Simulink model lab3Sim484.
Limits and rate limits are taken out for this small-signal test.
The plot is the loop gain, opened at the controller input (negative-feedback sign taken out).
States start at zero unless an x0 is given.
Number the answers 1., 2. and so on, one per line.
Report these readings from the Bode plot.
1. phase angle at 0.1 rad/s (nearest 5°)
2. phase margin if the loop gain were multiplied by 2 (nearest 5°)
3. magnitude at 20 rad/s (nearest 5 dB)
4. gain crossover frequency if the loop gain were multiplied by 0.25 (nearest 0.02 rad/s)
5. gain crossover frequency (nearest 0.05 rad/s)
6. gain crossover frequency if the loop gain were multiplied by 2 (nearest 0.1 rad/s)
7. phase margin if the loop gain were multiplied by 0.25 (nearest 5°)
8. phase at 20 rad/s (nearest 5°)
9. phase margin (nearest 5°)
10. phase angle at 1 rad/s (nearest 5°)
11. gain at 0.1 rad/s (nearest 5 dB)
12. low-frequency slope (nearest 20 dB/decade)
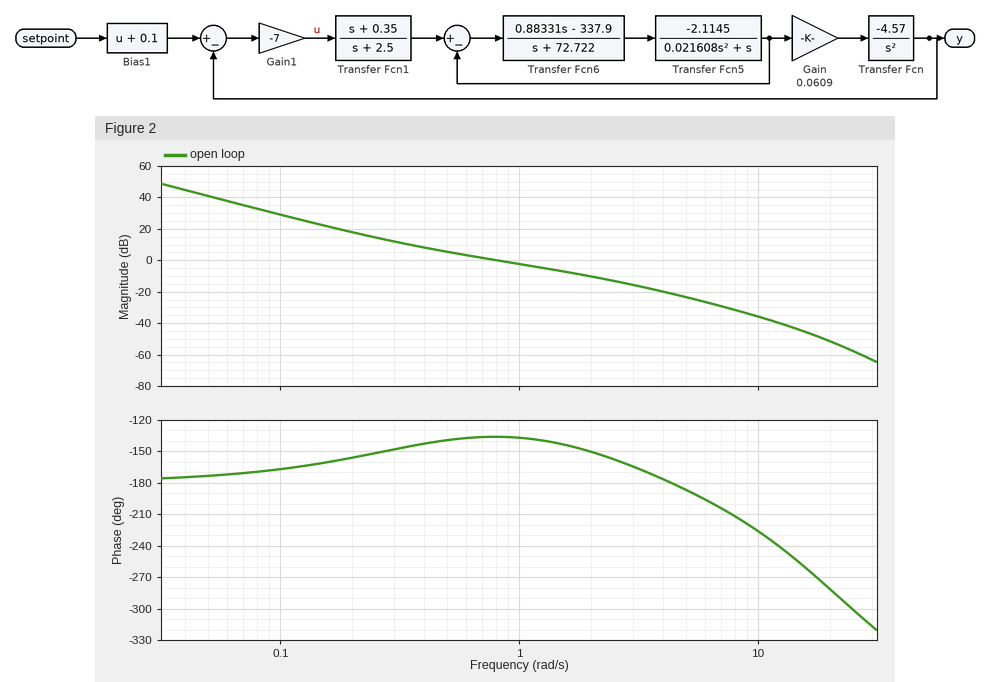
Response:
1. -165°
2. 40°
3. -50 dB
4. 0.30 rad/s
5. 0.80 rad/s
6. 1.4 rad/s
7. 30°
8. -280°
9. 45°
10. -135°
11. 30 dB
12. -40 dB/decade
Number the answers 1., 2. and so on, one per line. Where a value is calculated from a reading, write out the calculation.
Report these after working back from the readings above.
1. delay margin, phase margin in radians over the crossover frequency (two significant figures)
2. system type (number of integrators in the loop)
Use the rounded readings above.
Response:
1. 45 × π / 180 / 0.8 = 0.98 s
2. 2
